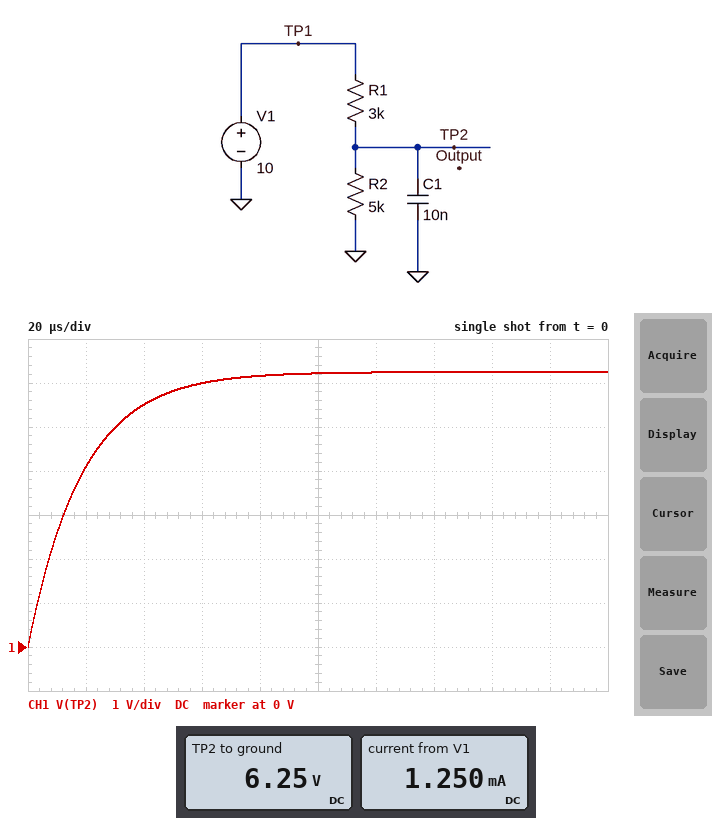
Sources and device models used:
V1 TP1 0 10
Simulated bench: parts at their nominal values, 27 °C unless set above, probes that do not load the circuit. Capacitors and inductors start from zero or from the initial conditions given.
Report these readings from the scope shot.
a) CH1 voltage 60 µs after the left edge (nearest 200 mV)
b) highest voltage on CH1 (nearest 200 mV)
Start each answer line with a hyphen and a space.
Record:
- 6.0 V
- 6.2 V
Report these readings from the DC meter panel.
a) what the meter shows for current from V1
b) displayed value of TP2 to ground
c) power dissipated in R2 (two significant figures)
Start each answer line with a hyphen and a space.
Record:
- 1.250 mA
- 6.25 V
- 7.8 mW
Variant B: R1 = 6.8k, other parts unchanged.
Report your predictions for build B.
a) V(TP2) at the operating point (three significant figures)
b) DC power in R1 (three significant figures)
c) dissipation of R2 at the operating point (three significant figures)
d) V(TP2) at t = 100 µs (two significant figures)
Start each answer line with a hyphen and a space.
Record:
- 4.24 V
- 4.88 mW
- 3.59 mW
- 4.1 V
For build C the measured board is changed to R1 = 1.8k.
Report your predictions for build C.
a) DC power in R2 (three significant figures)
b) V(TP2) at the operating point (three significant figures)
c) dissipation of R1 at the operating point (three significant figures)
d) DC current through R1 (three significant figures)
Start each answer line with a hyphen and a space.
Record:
- 10.8 mW
- 7.35 V
- 3.89 mW
- 1.47 mA
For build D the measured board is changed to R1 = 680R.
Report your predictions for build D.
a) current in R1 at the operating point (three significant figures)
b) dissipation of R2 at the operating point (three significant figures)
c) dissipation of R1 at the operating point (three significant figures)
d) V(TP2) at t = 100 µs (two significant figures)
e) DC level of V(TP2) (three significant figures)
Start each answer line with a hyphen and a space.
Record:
- 1.76 mA
- 15.5 mW
- 2.11 mW
- 8.8 V
- 8.80 V
